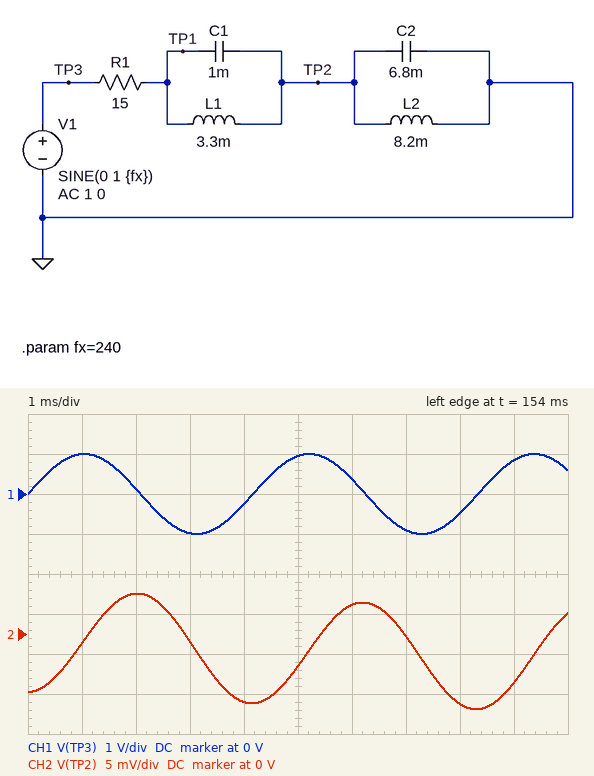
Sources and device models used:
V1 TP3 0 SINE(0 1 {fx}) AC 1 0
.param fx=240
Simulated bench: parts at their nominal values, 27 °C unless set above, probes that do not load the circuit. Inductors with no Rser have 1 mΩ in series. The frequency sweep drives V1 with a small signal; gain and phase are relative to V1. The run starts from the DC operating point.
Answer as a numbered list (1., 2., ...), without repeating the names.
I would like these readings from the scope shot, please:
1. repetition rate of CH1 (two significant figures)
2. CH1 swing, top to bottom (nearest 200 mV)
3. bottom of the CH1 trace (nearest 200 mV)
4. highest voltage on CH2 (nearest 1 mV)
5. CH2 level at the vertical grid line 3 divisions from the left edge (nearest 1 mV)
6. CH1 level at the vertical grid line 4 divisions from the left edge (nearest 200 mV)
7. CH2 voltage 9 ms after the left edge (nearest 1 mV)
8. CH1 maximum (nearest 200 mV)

1. 240 Hz
2. 2.0 V
3. -1.0 V
4. 5 mV
5. -1 mV
6. -200 mV
7. -6 mV
8. 1.0 V
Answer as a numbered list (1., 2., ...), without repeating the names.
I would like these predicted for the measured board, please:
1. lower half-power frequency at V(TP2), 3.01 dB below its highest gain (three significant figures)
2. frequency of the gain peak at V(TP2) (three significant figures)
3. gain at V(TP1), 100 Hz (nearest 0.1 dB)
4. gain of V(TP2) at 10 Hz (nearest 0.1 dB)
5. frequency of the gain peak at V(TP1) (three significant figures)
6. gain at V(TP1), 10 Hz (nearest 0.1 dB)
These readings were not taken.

1. 20.6 Hz
2. 21.3 Hz
3. -7.4 dB
4. -27.1 dB
5. 87.6 Hz
6. -24.7 dB
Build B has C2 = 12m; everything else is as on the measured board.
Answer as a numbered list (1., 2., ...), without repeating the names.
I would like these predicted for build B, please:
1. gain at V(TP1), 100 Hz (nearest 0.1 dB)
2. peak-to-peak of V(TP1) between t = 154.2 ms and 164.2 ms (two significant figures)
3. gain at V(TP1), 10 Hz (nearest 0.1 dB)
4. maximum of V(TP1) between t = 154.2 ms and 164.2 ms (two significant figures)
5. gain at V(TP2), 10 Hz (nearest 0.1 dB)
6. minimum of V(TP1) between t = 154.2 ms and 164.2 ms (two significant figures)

1. -7.5 dB
2. 110 mV
3. -23.1 dB
4. 53 mV
5. -25.0 dB
6. -57 mV
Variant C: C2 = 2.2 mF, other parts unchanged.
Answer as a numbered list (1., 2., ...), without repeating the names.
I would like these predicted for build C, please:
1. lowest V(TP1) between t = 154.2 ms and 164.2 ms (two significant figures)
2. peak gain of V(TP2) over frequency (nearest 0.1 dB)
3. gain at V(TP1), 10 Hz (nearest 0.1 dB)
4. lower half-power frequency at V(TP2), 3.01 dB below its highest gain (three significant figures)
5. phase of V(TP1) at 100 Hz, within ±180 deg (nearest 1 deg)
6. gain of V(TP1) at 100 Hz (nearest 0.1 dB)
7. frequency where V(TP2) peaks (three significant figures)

1. -71 mV
2. 0 dB
3. -25.9 dB
4. 35.3 Hz
5. -63 deg
6. -6.8 dB
7. 37.6 Hz
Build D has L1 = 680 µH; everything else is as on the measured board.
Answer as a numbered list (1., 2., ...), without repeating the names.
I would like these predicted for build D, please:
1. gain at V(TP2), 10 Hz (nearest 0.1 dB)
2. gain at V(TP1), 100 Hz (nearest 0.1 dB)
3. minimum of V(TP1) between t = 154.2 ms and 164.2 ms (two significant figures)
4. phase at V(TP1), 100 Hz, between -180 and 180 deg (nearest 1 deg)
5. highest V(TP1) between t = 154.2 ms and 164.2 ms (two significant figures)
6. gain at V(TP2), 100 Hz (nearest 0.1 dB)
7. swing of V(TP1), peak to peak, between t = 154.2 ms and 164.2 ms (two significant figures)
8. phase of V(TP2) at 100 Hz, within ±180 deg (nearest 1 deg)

1. -27.1 dB
2. -32.9 dB
3. -130 mV
4. 88 deg
5. 130 mV
6. -35.7 dB
7. 260 mV
8. -91 deg
